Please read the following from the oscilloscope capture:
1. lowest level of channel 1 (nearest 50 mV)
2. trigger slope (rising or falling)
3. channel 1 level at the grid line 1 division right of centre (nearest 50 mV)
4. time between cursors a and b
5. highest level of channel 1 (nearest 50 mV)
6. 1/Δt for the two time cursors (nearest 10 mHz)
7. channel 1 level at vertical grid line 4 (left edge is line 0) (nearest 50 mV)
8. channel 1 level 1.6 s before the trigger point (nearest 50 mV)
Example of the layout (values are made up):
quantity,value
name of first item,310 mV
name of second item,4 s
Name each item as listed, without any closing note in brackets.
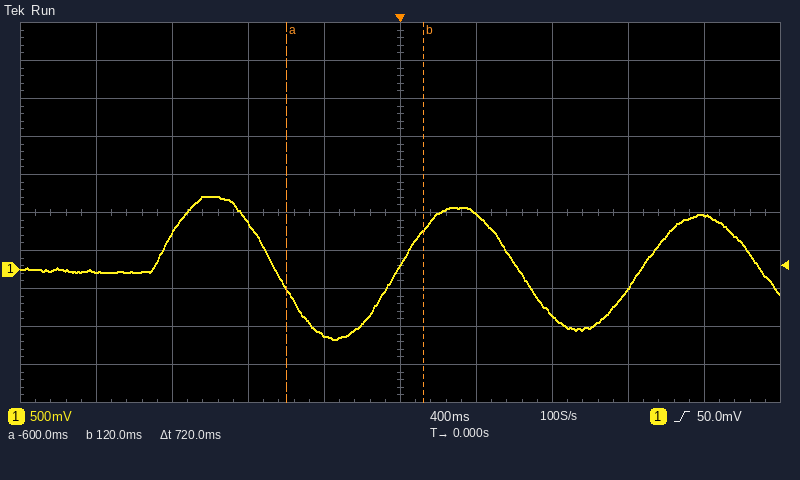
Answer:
quantity,value
lowest level of channel 1,-900 mV
trigger slope,rising
channel 1 level at the grid line 1 division right of centre,750 mV
time between cursors a and b,720 ms
highest level of channel 1,950 mV
1/Δt for the two time cursors,1.39 Hz
channel 1 level at vertical grid line 4 (left edge is line 0),-850 mV
channel 1 level 1.6 s before the trigger point,-50 mV
